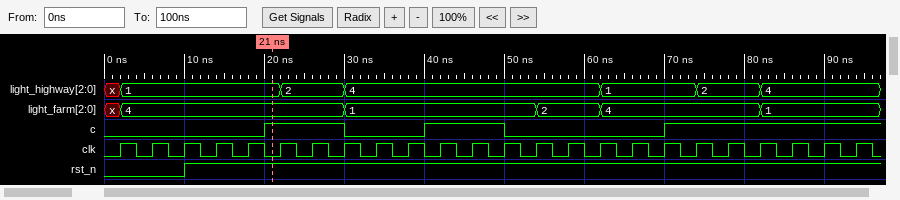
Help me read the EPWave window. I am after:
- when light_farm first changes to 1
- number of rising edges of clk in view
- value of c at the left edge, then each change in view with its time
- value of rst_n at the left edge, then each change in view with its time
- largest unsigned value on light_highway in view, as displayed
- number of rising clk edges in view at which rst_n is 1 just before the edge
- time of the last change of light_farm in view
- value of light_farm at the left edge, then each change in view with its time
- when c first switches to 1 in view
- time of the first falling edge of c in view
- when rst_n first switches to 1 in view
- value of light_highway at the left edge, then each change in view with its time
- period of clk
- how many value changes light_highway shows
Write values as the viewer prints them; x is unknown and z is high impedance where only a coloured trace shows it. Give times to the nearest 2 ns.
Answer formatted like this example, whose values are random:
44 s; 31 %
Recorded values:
30 ns; 24; 0, 1 at 20 ns, 0 at 30 ns, 1 at 40 ns, 0 at 50 ns, 1 at 70 ns; 0, 1 at 10 ns; 4; 21; 82 ns; x, 4 at 2 ns, 1 at 30 ns, 2 at 54 ns, 4 at 62 ns, 1 at 82 ns; 20 ns; 30 ns; 10 ns; x, 1 at 2 ns, 2 at 22 ns, 4 at 30 ns, 1 at 62 ns, 2 at 74 ns, 4 at 82 ns; 4 ns; 6
